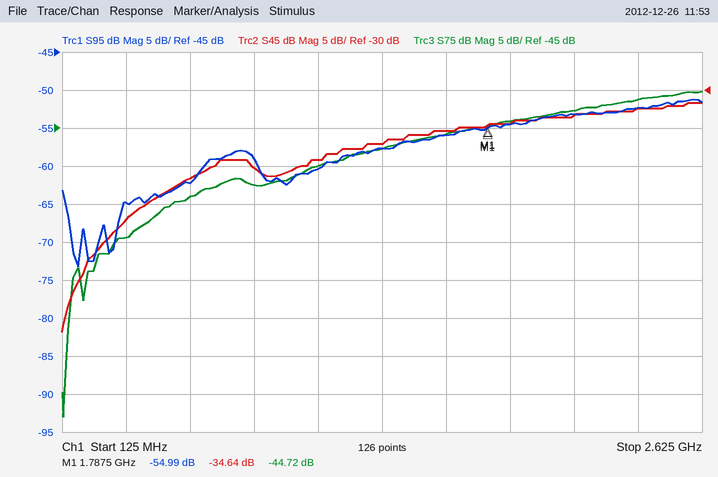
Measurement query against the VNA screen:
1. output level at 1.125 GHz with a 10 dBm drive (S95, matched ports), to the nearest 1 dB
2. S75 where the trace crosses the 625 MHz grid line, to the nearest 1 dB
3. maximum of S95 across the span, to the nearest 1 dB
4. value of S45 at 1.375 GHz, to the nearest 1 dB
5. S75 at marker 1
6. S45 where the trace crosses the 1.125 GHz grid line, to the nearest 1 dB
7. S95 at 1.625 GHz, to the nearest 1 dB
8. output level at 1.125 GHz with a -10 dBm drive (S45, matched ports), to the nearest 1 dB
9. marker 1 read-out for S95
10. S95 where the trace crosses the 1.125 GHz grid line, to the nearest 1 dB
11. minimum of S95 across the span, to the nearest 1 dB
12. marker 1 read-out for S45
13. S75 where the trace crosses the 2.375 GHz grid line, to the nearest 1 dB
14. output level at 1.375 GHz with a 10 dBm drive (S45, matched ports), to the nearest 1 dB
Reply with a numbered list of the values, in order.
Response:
1. -50 dBm
2. -54 dB
3. -51 dB
4. -37 dB
5. -44.72 dB
6. -39 dB
7. -56 dB
8. -49 dBm
9. -54.99 dB
10. -60 dB
11. -73 dB
12. -34.64 dB
13. -41 dB
14. -27 dBm
